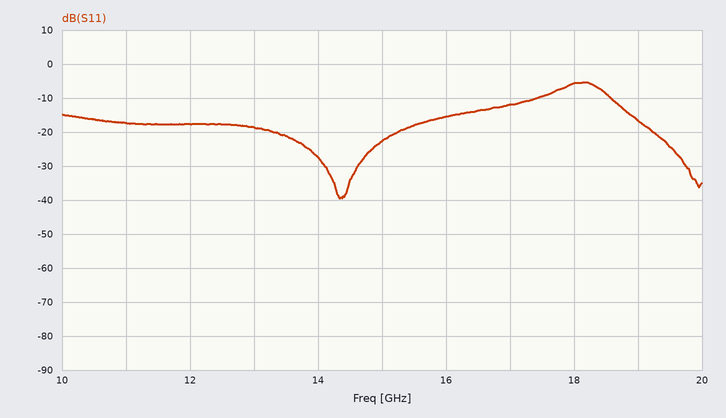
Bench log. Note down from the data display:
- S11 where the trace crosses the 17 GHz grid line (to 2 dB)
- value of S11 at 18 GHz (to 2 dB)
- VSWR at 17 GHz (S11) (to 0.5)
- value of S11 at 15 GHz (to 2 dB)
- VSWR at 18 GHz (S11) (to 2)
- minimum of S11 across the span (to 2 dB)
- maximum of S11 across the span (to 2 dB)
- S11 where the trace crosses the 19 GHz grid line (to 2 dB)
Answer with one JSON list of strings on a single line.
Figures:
["-12 dB", "-6 dB", "1.5", "-22 dB", "4", "-40 dB", "-6 dB", "-16 dB"]
